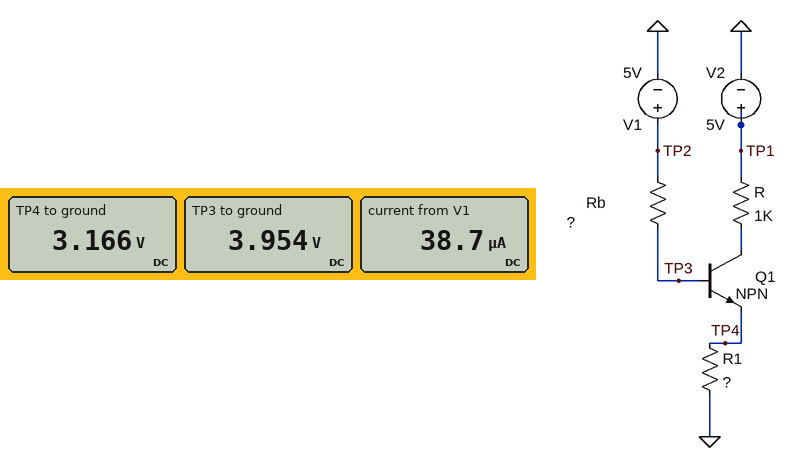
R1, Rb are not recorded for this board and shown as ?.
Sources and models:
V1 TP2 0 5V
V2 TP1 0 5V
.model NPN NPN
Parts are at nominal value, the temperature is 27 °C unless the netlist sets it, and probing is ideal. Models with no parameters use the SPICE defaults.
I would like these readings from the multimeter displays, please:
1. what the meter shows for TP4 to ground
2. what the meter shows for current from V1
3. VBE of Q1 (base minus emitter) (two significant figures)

3.166 V
38.7 µA
790 mV
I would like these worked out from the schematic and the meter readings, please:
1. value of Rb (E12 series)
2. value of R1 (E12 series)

27 kΩ
1.8 kΩ
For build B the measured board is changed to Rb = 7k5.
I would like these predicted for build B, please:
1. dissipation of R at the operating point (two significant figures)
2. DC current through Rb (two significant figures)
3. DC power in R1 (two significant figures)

2.8 mW
130 µA
5.9 mW
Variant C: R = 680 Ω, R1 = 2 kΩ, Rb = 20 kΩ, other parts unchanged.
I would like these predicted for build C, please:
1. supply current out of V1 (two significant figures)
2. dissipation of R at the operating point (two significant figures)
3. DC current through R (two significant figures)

28 µA
2.2 mW
1.8 mA
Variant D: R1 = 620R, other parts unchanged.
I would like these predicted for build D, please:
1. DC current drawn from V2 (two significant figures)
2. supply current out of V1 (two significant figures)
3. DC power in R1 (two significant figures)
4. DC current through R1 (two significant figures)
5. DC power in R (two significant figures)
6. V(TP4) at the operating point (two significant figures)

3.0 mA
85 µA
5.9 mW
3.1 mA
8.9 mW
1.9 V
